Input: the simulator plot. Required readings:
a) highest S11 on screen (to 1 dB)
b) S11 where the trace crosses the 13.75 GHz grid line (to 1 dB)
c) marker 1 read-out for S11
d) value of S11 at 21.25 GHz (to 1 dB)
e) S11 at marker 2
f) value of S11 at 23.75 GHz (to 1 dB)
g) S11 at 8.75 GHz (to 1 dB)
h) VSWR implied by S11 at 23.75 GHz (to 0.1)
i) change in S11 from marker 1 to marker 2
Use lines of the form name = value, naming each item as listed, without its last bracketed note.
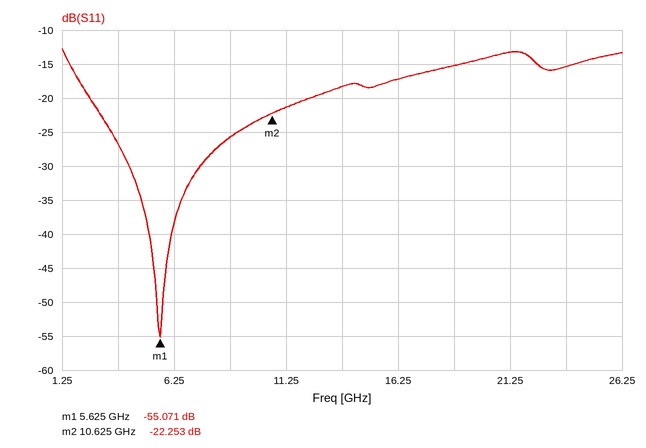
highest S11 on screen = -13 dB
S11 where the trace crosses the 13.75 GHz grid line = -18 dB
marker 1 read-out for S11 = -55.071 dB
value of S11 at 21.25 GHz = -13 dB
S11 at marker 2 = -22.253 dB
value of S11 at 23.75 GHz = -15 dB
S11 at 8.75 GHz = -26 dB
VSWR implied by S11 at 23.75 GHz = 1.4
change in S11 from marker 1 to marker 2 = 32.818 dB
